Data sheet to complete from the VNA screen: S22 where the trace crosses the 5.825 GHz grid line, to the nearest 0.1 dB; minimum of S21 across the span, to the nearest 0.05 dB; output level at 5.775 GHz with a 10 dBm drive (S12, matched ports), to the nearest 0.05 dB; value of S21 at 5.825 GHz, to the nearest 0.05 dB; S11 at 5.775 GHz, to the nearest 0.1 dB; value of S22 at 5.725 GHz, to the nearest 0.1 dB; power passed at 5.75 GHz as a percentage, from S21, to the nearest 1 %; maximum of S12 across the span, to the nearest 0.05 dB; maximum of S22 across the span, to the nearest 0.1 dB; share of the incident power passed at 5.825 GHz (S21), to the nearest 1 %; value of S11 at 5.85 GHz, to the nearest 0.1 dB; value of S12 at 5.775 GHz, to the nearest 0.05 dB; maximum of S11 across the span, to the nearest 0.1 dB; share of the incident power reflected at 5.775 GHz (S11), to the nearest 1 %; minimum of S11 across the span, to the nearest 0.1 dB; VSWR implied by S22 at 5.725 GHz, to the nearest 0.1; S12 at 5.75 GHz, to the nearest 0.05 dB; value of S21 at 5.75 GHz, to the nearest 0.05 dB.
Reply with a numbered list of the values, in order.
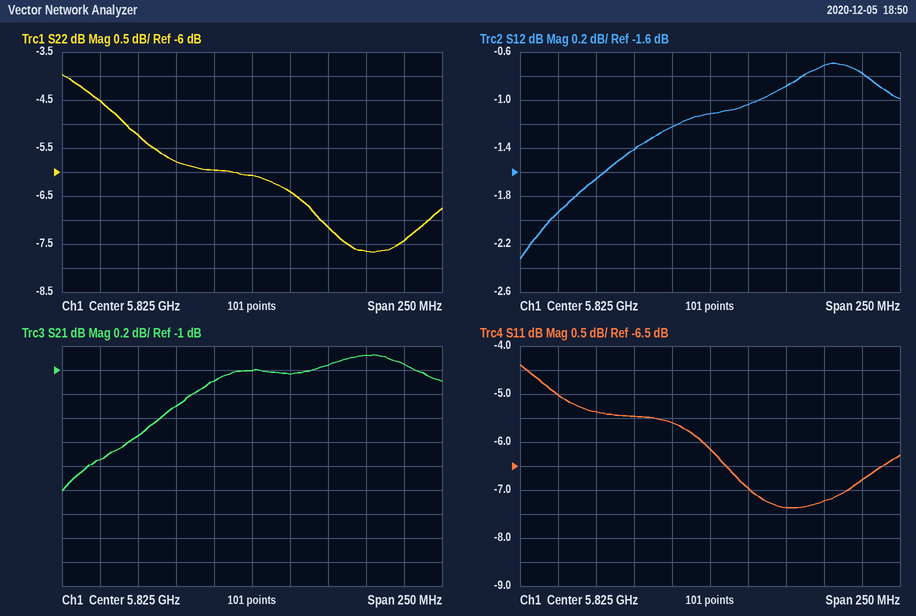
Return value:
1. -6.1 dB
2. -2.00 dB
3. 8.60 dBm
4. -1.00 dB
5. -5.5 dB
6. -4.5 dB
7. 70 %
8. -0.70 dB
9. -4.0 dB
10. 79 %
11. -7.0 dB
12. -1.40 dB
13. -4.4 dB
14. 28 %
15. -7.4 dB
16. 3.9
17. -1.65 dB
18. -1.55 dB
